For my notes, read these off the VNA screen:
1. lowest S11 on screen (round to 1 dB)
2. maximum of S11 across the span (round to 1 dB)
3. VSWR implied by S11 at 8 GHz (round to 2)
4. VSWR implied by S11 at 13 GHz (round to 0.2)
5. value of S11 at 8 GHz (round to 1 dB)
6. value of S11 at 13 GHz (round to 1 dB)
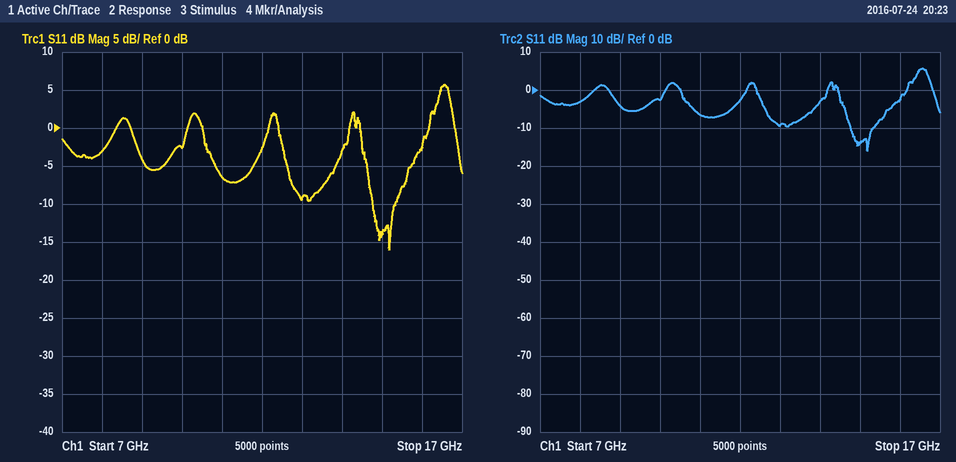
-16 dB
6 dB
6
2.0
-3 dB
-9 dB
